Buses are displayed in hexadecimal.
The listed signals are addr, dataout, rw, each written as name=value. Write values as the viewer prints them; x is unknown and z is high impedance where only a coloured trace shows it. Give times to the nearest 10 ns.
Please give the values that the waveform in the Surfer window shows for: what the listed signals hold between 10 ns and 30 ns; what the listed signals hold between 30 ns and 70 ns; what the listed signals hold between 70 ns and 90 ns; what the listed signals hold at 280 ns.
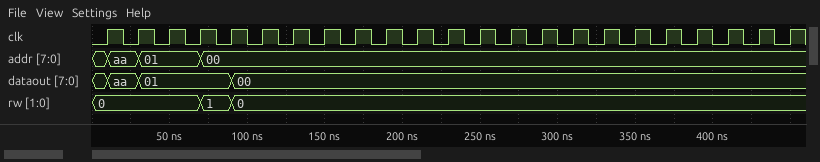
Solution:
addr=aa, dataout=aa, rw=0
addr=01, dataout=01, rw=0
addr=00, dataout=01, rw=1
addr=00, dataout=00, rw=0
